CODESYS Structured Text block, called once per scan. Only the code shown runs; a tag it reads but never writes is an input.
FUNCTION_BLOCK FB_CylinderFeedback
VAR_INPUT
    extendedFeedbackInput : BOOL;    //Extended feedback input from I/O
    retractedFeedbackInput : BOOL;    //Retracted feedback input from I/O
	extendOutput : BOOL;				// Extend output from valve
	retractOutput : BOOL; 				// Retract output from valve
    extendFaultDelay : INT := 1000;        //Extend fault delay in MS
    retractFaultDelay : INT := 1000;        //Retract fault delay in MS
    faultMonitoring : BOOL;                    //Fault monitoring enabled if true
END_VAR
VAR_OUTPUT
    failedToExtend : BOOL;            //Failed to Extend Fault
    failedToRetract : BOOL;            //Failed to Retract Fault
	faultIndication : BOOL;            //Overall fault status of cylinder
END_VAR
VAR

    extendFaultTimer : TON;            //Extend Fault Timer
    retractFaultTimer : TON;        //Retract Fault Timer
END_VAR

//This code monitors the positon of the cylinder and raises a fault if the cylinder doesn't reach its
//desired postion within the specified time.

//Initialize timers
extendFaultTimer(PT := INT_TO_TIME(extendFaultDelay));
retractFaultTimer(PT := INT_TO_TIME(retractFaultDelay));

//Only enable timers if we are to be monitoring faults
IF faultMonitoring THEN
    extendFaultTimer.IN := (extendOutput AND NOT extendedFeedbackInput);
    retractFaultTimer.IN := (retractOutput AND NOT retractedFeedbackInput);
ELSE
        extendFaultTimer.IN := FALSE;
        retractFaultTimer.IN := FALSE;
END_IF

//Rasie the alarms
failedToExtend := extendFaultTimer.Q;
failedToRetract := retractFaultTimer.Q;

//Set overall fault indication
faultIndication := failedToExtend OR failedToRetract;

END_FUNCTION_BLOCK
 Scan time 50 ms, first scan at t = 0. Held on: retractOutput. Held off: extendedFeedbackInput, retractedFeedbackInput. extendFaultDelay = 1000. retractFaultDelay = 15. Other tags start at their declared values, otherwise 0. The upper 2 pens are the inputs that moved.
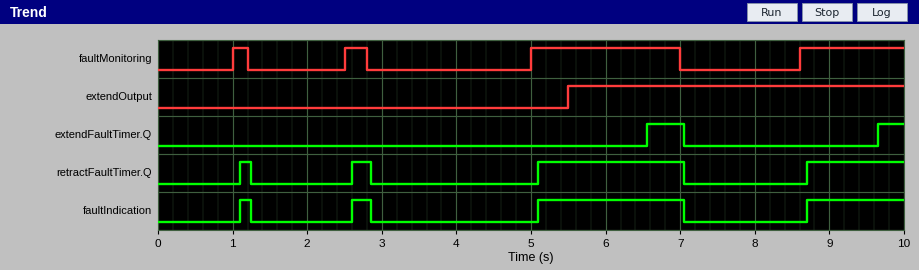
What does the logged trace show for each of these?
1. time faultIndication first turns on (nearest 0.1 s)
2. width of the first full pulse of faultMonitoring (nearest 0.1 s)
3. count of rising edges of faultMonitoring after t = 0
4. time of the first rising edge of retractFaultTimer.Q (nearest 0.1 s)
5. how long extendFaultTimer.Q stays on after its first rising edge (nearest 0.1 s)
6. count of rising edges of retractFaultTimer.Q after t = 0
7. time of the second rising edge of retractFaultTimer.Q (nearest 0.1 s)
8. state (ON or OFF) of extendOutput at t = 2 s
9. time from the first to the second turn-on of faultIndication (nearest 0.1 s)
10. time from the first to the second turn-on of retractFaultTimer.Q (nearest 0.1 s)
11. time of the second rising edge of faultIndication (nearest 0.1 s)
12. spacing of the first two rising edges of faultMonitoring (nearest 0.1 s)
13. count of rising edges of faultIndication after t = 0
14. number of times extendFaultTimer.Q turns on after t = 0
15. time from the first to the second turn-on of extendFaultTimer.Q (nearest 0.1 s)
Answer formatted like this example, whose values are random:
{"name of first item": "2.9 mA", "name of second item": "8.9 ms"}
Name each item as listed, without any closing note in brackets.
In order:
{"time faultIndication first turns on": "1.1 s", "width of the first full pulse of faultMonitoring": "0.2 s", "count of rising edges of faultMonitoring after t = 0": "4", "time of the first rising edge of retractFaultTimer.Q": "1.1 s", "how long extendFaultTimer.Q stays on after its first rising edge": "0.5 s", "count of rising edges of retractFaultTimer.Q after t = 0": "4", "time of the second rising edge of retractFaultTimer.Q": "2.6 s", "state (ON or OFF) of extendOutput at t = 2 s": "OFF", "time from the first to the second turn-on of faultIndication": "1.5 s", "time from the first to the second turn-on of retractFaultTimer.Q": "1.5 s", "time of the second rising edge of faultIndication": "2.6 s", "spacing of the first two rising edges of faultMonitoring": "1.5 s", "count of rising edges of faultIndication after t = 0": "4", "number of times extendFaultTimer.Q turns on after t = 0": "2", "time from the first to the second turn-on of extendFaultTimer.Q": "3.1 s"}
